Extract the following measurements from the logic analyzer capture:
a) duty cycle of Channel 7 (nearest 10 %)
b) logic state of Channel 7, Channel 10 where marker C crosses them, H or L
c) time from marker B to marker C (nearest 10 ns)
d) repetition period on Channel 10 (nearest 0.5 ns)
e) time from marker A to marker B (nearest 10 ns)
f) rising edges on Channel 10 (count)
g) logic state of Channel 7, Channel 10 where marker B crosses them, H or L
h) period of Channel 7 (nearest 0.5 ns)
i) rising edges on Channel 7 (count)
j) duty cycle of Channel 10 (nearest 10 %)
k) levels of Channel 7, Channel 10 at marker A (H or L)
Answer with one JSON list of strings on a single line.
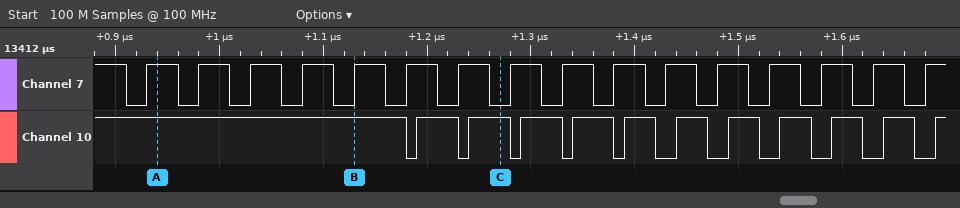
["60 %", "Channel 7=L, Channel 10=H", "140 ns", "50 ns", "190 ns", "11", "Channel 7=H, Channel 10=H", "50 ns", "16", "70 %", "Channel 7=H, Channel 10=H"]
